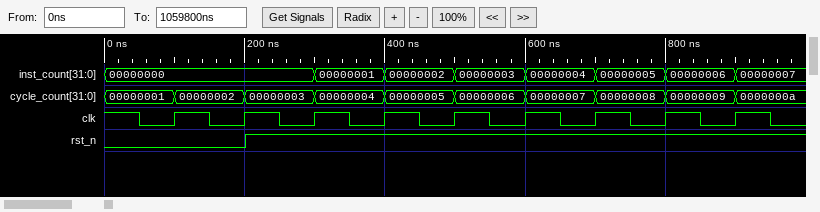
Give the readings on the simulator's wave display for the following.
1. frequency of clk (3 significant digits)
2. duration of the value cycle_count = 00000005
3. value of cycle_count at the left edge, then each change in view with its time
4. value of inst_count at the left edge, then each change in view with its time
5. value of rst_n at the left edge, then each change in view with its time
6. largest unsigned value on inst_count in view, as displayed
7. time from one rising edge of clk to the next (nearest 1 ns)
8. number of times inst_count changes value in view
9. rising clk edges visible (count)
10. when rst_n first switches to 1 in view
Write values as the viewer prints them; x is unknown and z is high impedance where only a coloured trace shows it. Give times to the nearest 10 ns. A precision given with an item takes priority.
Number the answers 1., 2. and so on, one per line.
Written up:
1. 10.0 MHz
2. 100 ns
3. 00000001, 00000002 at 100 ns, 00000003 at 200 ns, 00000004 at 300 ns, 00000005 at 400 ns, 00000006 at 500 ns, 00000007 at 600 ns, 00000008 at 700 ns, 00000009 at 800 ns, 0000000a at 900 ns
4. 00000000, 00000001 at 300 ns, 00000002 at 400 ns, 00000003 at 500 ns, 00000004 at 600 ns, 00000005 at 700 ns, 00000006 at 800 ns, 00000007 at 900 ns
5. 0, 1 at 200 ns
6. 00000007
7. 100 ns
8. 7
9. 9
10. 200 ns
